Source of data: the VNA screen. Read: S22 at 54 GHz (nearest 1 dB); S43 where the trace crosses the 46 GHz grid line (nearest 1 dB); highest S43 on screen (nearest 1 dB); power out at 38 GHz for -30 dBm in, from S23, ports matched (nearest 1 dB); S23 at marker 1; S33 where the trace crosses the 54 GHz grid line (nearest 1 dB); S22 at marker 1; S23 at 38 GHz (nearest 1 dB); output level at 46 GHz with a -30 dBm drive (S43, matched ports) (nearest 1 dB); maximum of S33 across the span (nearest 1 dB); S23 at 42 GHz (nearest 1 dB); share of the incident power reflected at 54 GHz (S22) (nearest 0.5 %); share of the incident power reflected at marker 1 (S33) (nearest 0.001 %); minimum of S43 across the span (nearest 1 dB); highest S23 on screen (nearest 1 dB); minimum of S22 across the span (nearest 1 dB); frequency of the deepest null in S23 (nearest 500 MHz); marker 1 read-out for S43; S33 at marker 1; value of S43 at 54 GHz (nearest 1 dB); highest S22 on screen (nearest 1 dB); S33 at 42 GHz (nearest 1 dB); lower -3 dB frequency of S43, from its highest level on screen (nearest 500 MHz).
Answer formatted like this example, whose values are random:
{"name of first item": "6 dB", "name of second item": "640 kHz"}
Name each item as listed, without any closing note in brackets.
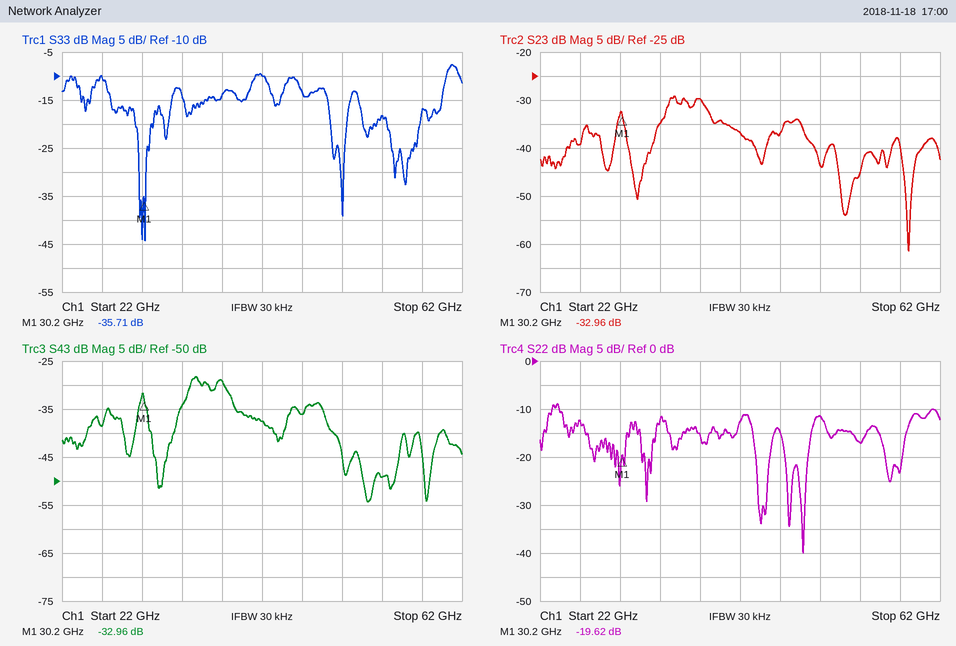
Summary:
{"S22 at 54 GHz": "-17 dB", "S43 where the trace crosses the 46 GHz grid line": "-36 dB", "highest S43 on screen": "-28 dB", "power out at 38 GHz for -30 dBm in, from S23, ports matched": "-60 dBm", "S23 at marker 1": "-32.96 dB", "S33 where the trace crosses the 54 GHz grid line": "-18 dB", "S22 at marker 1": "-19.62 dB", "S23 at 38 GHz": "-30 dB", "output level at 46 GHz with a -30 dBm drive (S43, matched ports)": "-66 dBm", "maximum of S33 across the span": "-8 dB", "S23 at 42 GHz": "-37 dB", "share of the incident power reflected at 54 GHz (S22)": "2.0 %", "share of the incident power reflected at marker 1 (S33)": "0.027 %", "minimum of S43 across the span": "-54 dB", "highest S23 on screen": "-29 dB", "minimum of S22 across the span": "-40 dB", "frequency of the deepest null in S23": "59.0 GHz", "marker 1 read-out for S43": "-32.96 dB", "S33 at marker 1": "-35.71 dB", "value of S43 at 54 GHz": "-49 dB", "highest S22 on screen": "-9 dB", "S33 at 42 GHz": "-10 dB", "lower -3 dB frequency of S43, from its highest level on screen": "34.5 GHz"}
